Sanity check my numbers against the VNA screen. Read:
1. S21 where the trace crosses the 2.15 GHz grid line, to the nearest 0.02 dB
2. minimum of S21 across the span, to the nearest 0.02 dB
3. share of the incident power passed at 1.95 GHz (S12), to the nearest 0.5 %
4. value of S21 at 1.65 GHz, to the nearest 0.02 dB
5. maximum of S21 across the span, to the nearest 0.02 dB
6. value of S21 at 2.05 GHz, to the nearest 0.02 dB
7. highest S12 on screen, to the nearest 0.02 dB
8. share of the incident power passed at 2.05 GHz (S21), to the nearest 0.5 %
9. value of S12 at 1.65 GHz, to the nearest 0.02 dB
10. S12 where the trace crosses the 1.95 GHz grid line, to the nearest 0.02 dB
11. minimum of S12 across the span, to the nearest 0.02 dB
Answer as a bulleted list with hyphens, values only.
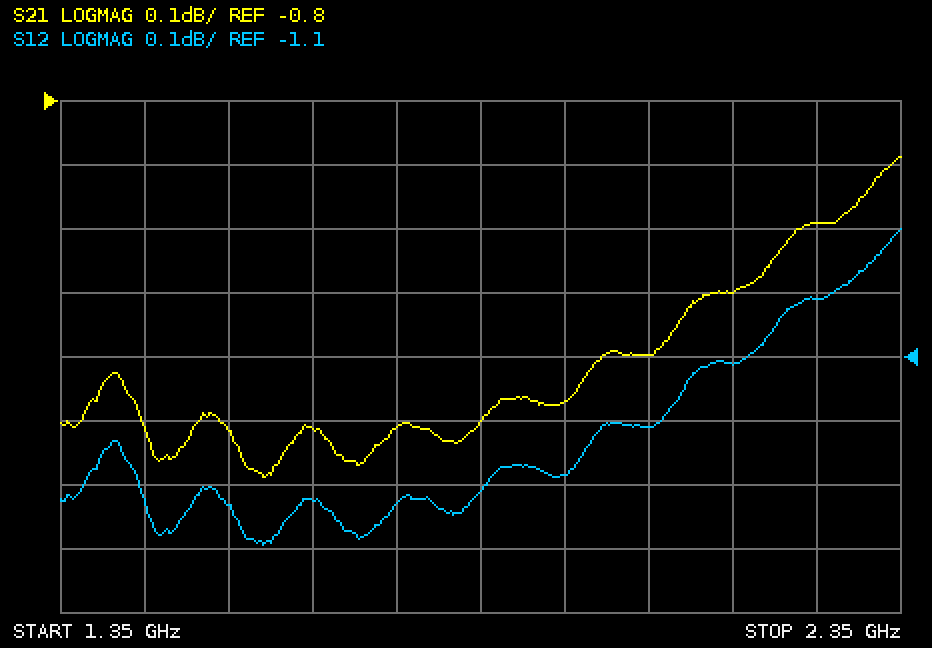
- -1.10 dB
- -1.38 dB
- 74.5 %
- -1.32 dB
- -0.88 dB
- -1.20 dB
- -0.90 dB
- 76.0 %
- -1.32 dB
- -1.28 dB
- -1.40 dB
